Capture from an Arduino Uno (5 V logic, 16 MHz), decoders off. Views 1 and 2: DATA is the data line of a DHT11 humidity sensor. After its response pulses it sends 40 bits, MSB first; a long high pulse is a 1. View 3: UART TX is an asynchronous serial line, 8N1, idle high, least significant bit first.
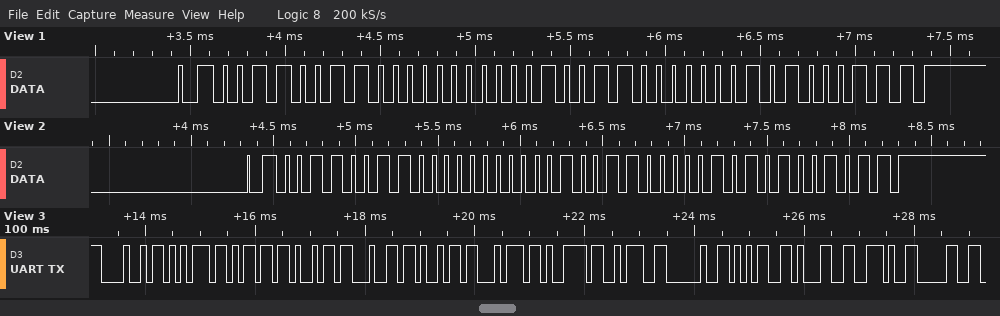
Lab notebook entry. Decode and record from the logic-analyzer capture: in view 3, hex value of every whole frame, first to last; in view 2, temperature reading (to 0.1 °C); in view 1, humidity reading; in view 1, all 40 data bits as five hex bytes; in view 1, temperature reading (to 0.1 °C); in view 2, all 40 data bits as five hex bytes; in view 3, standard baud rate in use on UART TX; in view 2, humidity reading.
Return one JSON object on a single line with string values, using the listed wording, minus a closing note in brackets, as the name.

{"in view 3, hex value of every whole frame, first to last": "0x48 0x75 0x6D 0x69 0x64 0x69 0x74 0x79 0x3A 0x20 0x35 0x31 0x2E 0x30", "in view 2, temperature reading": "19.5 °C", "in view 1, humidity reading": "51 %", "in view 1, all 40 data bits as five hex bytes": "33 00 13 01 47", "in view 1, temperature reading": "19.1 °C", "in view 2, all 40 data bits as five hex bytes": "33 00 13 05 4B", "in view 3, standard baud rate in use on UART TX": "9600 baud", "in view 2, humidity reading": "51 %"}
